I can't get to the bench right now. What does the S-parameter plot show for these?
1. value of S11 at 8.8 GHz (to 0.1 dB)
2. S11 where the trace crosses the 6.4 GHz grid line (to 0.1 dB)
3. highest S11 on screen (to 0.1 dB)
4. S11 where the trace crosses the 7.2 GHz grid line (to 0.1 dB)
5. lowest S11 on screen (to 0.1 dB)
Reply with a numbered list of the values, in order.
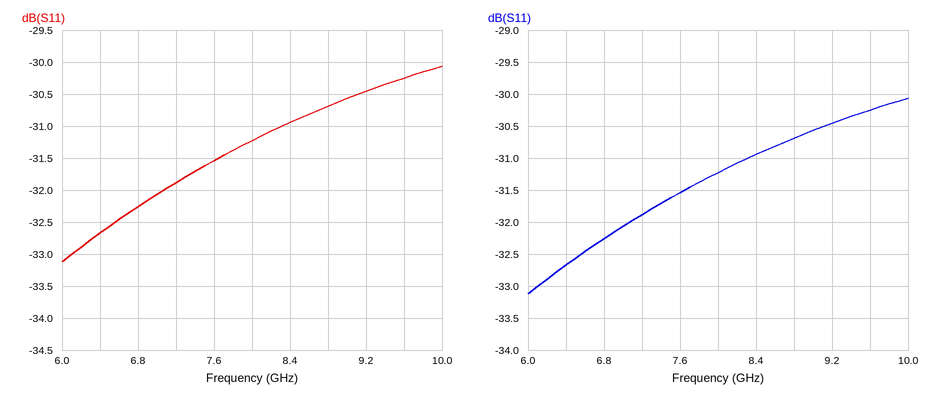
1. -30.7 dB
2. -32.7 dB
3. -30.1 dB
4. -31.9 dB
5. -33.1 dB
